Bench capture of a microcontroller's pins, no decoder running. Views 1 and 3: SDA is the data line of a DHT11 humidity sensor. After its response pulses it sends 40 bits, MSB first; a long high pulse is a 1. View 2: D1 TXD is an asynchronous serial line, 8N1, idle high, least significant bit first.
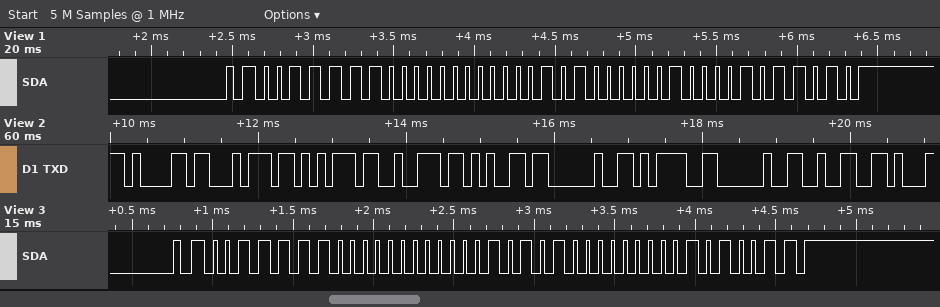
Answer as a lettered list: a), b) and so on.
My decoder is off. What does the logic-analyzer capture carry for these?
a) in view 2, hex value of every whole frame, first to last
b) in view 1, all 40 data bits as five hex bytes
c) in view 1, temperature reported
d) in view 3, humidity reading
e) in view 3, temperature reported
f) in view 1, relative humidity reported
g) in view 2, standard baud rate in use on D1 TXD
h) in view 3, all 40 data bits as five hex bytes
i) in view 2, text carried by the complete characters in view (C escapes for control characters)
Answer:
a) 61 74 75 72 65 20 3D 20 32
b) 3E 00 14 08 5A
c) 20.8 °C
d) 62 %
e) 21.0 °C
f) 62 %
g) 9600 baud
h) 3E 00 15 00 53
i) "ature = 2"
